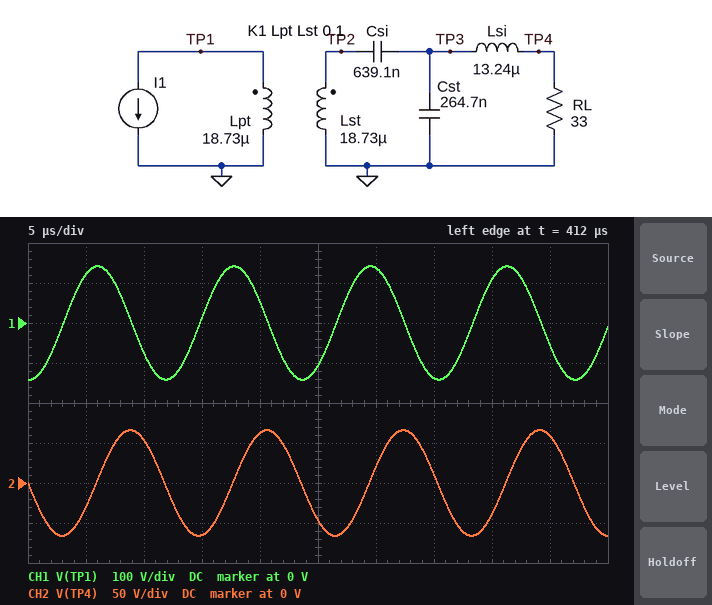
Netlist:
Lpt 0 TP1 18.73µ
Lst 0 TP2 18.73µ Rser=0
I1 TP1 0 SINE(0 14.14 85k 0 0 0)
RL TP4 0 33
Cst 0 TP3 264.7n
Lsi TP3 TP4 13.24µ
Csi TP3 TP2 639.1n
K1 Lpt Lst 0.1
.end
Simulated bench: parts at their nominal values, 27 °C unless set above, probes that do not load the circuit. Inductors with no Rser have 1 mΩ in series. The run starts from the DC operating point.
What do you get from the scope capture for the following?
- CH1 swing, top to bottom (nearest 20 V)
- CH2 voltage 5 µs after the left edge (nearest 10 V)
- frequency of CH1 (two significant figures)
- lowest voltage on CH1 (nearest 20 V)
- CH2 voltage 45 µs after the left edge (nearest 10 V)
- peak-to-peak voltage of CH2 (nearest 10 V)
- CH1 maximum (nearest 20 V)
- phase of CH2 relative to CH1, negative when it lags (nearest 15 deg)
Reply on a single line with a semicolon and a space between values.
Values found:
280 V; -30 V; 85 kHz; -140 V; 60 V; 130 V; 140 V; -90 deg
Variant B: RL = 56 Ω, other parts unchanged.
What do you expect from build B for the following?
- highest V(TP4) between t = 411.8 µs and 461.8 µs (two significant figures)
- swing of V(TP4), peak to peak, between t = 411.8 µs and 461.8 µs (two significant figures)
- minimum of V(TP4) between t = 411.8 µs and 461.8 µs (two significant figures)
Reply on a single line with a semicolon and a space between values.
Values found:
110 V; 220 V; -110 V
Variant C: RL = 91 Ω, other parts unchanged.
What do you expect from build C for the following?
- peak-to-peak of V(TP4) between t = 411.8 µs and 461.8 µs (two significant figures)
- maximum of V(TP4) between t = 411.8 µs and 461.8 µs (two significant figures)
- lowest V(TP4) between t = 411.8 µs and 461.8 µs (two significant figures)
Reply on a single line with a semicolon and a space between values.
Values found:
360 V; 180 V; -180 V
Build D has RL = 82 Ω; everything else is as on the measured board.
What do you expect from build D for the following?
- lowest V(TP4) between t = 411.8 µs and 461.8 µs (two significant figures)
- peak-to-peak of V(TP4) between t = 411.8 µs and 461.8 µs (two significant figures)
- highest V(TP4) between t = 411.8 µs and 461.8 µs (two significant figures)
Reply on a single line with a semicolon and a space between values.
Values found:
-160 V; 330 V; 160 V
